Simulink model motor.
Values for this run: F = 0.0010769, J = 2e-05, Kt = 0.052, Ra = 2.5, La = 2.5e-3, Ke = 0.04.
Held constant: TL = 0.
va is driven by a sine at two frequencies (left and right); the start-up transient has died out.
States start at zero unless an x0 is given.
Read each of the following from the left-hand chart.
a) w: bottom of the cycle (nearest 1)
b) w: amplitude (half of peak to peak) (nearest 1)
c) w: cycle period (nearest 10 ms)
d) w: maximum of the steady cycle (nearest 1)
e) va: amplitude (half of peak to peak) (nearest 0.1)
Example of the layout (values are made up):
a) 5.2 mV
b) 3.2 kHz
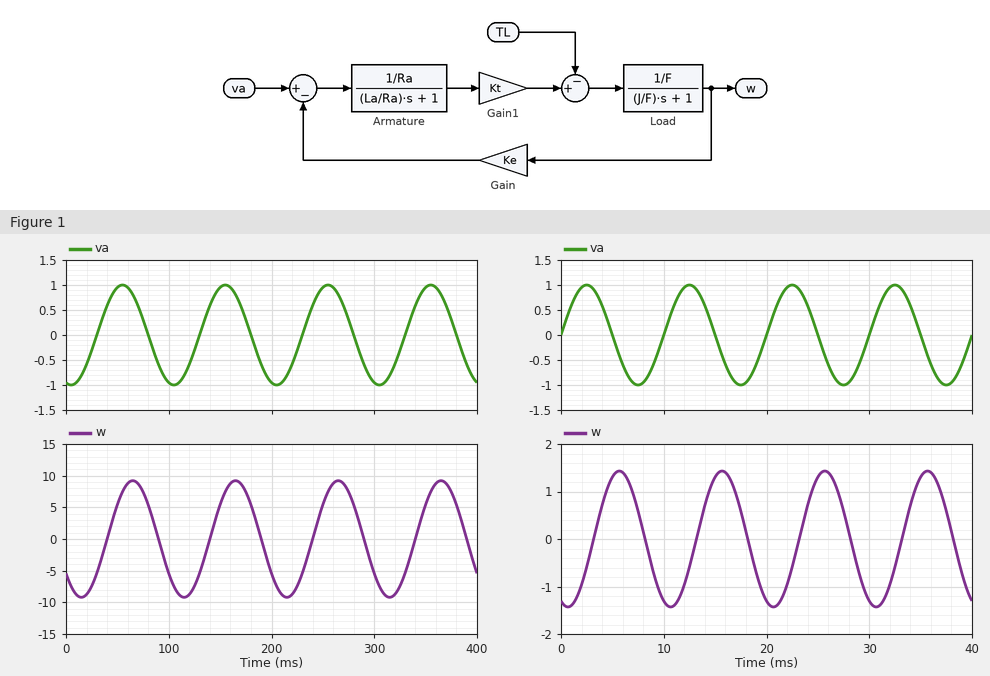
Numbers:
a) -9
b) 9
c) 100 ms
d) 9
e) 1.0
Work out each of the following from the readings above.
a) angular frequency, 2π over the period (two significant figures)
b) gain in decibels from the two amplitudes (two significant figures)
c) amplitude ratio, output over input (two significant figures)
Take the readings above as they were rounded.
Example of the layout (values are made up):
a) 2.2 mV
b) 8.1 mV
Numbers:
a) 0.063 rad/ms
b) 19 dB
c) 9.0
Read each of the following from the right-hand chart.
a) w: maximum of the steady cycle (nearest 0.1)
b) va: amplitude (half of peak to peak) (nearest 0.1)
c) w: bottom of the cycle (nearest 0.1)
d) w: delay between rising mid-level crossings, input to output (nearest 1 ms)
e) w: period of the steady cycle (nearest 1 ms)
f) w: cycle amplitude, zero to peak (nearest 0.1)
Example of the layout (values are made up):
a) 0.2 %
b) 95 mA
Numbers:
a) 1.4
b) 1.0
c) -1.4
d) 3 ms
e) 10 ms
f) 1.4
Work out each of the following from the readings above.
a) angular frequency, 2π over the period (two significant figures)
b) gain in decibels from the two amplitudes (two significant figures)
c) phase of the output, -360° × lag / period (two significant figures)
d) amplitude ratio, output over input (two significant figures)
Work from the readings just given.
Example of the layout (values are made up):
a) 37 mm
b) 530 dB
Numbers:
a) 0.63 rad/ms
b) 2.9 dB
c) -110°
d) 1.4
